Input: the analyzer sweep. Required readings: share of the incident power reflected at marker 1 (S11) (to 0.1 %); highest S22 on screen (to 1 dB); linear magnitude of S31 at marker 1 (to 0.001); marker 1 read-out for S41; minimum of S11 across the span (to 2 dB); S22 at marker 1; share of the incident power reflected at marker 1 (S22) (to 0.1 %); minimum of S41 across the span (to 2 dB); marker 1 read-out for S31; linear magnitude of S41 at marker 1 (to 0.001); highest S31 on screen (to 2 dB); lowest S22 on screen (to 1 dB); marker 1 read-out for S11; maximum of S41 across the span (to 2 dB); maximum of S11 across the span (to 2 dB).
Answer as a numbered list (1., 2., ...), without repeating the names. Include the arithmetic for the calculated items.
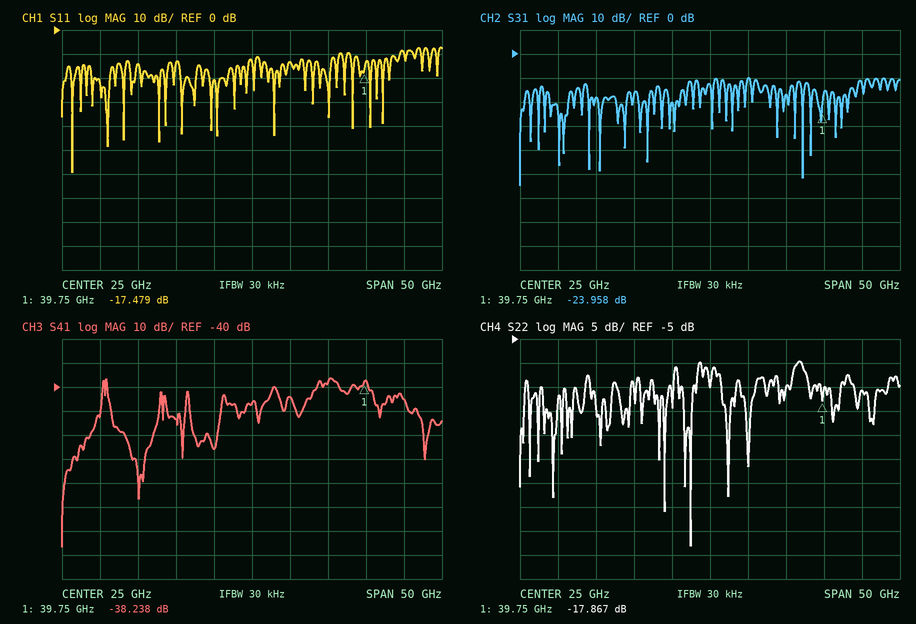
1. 10^(-17.479/10) ≈ 1.8 %
2. -10 dB
3. 10^(-23.958/20) ≈ 0.063
4. -38.238 dB
5. -60 dB
6. -17.867 dB
7. 10^(-17.867/10) ≈ 1.6 %
8. -106 dB
9. -23.958 dB
10. 10^(-38.238/20) ≈ 0.012
11. -10 dB
12. -48 dB
13. -17.479 dB
14. -36 dB
15. -8 dB
